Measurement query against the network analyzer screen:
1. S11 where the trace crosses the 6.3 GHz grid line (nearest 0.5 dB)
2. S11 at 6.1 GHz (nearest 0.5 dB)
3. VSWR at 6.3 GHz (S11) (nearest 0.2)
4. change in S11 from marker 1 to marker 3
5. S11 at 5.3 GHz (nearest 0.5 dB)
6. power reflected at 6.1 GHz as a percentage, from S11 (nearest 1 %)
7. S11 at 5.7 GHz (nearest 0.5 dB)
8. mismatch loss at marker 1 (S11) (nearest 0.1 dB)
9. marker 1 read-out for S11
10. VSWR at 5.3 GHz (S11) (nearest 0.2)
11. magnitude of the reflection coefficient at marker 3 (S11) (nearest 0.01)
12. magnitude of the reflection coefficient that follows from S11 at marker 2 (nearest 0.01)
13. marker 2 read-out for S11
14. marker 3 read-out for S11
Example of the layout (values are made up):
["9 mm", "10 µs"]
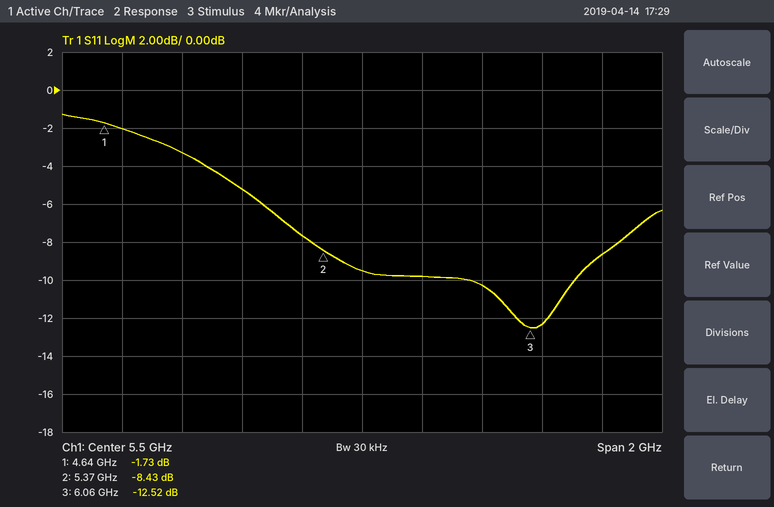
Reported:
["-8.5 dB", "-12.5 dB", "2.2", "-10.79 dB", "-7.5 dB", "6 %", "-10.0 dB", "4.8 dB", "-1.73 dB", "2.4", "0.24", "0.38", "-8.43 dB", "-12.52 dB"]
